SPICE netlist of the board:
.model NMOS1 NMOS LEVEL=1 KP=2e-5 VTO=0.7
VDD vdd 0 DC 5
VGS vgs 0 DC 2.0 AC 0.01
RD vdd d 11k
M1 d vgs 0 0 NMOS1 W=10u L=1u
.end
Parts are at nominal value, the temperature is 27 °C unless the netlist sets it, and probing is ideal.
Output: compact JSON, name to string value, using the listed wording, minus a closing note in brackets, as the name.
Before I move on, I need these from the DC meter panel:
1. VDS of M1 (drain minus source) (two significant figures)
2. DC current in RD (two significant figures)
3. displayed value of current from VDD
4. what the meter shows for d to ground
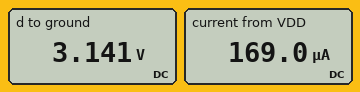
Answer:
{"VDS of M1 (drain minus source)": "3.1 V", "DC current in RD": "170 µA", "displayed value of current from VDD": "169.0 µA", "what the meter shows for d to ground": "3.141 V"}
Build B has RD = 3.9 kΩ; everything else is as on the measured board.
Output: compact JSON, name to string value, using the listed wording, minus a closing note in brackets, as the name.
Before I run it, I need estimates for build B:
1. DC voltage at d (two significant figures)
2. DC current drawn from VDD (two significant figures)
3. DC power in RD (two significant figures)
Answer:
{"DC voltage at d": "4.3 V", "DC current drawn from VDD": "170 µA", "DC power in RD": "110 µW"}
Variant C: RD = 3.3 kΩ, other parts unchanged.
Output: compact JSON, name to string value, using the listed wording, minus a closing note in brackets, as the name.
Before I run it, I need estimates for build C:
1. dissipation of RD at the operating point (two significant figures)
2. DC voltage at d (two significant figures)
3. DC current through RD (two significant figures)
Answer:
{"dissipation of RD at the operating point": "94 µW", "DC voltage at d": "4.4 V", "DC current through RD": "170 µA"}
